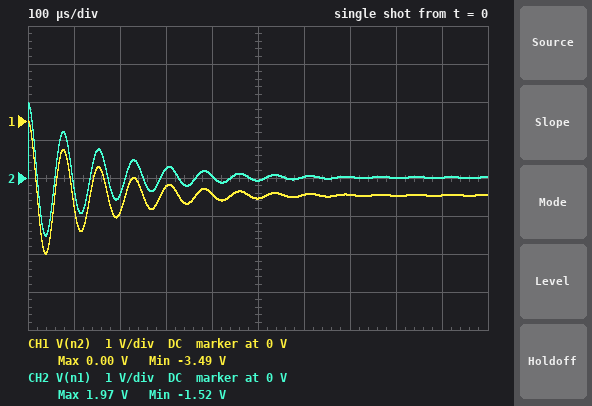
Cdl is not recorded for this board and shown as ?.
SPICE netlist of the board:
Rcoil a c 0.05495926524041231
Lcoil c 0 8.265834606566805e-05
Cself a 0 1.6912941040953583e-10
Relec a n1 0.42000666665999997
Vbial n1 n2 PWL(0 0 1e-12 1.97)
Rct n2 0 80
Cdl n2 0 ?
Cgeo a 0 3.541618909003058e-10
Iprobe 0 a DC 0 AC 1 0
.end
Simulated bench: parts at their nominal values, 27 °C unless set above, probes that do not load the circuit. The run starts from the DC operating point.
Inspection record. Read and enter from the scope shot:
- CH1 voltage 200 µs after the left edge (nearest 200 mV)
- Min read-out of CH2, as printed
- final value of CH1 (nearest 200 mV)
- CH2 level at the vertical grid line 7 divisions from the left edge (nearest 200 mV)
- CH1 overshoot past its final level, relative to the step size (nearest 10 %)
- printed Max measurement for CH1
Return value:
-2.4 V
-1.52 V
-2.0 V
0 V
80 %
0.00 V
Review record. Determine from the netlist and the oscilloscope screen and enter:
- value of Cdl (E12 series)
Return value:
1.8 µF
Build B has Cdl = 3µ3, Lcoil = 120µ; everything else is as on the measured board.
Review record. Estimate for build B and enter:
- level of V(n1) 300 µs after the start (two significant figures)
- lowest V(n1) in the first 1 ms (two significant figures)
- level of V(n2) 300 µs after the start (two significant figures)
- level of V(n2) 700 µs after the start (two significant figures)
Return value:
-450 mV
-1.5 V
-2.4 V
-2.1 V
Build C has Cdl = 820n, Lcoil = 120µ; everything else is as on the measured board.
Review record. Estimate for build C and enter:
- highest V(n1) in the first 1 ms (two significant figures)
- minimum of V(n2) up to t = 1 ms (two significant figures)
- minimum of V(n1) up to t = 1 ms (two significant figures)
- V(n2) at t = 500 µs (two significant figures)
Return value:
2.0 V
-3.4 V
-1.4 V
-1.9 V
